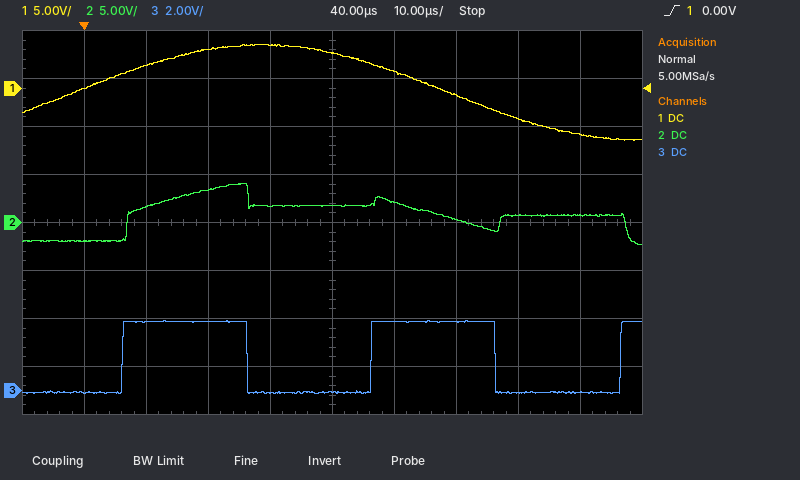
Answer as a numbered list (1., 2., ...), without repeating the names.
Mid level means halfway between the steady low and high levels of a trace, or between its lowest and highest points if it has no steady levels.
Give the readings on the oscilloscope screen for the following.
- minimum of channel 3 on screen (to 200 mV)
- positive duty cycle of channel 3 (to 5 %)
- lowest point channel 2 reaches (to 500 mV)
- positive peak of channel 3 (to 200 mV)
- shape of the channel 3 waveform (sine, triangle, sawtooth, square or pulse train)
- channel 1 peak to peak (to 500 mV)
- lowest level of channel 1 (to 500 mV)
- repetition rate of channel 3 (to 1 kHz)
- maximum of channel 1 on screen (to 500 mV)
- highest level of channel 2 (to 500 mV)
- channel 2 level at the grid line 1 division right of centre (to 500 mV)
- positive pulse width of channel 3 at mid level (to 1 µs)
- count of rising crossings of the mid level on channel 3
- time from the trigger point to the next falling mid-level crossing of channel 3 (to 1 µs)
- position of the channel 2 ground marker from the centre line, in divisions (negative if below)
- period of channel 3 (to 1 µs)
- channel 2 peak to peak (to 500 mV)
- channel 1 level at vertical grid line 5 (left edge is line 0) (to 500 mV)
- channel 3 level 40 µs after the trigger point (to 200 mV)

1. -200 mV
2. 50 %
3. -2.5 V
4. 3.0 V
5. square
6. 10.0 V
7. -5.5 V
8. 25 kHz
9. 4.5 V
10. 4.0 V
11. 2.0 V
12. 20 µs
13. 3
14. 26 µs
15. 0.0 div
16. 40 µs
17. 6.5 V
18. 3.5 V
19. 0.0 V
